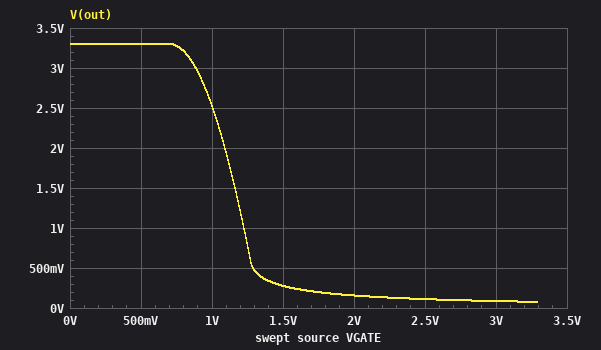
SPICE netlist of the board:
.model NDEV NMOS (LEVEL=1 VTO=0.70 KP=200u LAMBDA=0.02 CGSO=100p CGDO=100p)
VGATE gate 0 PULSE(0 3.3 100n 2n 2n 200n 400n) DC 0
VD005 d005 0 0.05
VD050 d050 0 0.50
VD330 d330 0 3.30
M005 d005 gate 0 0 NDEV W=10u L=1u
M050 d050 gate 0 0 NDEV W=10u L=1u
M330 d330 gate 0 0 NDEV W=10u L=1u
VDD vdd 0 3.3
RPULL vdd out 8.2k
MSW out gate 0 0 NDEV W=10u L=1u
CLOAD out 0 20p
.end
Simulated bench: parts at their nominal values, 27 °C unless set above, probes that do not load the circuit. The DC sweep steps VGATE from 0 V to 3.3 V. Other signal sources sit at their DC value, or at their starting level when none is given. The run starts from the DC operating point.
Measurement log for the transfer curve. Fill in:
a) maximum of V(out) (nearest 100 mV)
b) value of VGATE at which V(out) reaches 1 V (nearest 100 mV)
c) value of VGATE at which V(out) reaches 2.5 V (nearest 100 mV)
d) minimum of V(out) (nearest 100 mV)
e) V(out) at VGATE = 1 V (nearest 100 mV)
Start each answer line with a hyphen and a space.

- 3.3 V
- 1.2 V
- 1.0 V
- 100 mV
- 2.5 V
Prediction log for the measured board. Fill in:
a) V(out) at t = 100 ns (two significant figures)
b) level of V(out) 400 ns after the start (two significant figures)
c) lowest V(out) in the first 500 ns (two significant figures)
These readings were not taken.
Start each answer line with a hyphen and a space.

- 3.3 V
- 1.5 V
- 77 mV
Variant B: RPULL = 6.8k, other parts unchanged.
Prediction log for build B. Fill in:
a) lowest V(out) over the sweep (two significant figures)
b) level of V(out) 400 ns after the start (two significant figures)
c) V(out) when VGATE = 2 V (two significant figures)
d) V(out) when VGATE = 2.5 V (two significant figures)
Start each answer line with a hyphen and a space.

- 92 mV
- 1.7 V
- 190 mV
- 130 mV
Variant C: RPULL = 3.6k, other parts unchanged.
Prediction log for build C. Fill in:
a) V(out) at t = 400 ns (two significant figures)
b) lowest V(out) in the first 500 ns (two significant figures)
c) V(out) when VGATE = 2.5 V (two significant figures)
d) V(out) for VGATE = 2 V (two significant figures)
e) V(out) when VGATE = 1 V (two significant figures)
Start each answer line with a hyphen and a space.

- 2.5 V
- 170 mV
- 250 mV
- 360 mV
- 3.0 V
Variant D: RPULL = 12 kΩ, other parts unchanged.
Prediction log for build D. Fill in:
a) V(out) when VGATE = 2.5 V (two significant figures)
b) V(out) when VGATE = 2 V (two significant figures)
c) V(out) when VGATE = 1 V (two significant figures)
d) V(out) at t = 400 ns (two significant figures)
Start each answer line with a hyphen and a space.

- 76 mV
- 110 mV
- 2.2 V
- 1.1 V
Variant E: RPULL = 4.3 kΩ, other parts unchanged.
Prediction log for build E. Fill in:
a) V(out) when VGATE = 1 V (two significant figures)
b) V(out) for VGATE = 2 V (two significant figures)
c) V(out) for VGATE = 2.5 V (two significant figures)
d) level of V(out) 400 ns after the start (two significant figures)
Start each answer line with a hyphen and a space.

- 2.9 V
- 300 mV
- 210 mV
- 2.3 V
